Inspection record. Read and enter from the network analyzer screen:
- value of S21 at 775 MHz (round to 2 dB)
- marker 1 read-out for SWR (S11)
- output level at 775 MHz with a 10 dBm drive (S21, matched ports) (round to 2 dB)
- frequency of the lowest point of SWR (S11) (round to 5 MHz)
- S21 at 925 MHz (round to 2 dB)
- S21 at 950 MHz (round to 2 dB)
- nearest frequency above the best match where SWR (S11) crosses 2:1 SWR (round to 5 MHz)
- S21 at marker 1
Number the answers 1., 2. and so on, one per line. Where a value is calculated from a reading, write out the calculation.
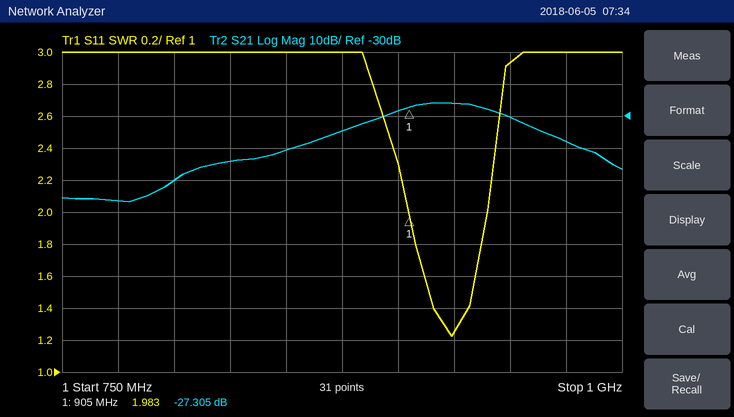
1. -56 dB
2. 1.983
3. 10 dBm + (-56 dB) = -46 dBm
4. 925 MHz
5. -26 dB
6. -30 dB
7. 940 MHz
8. -27.305 dB
